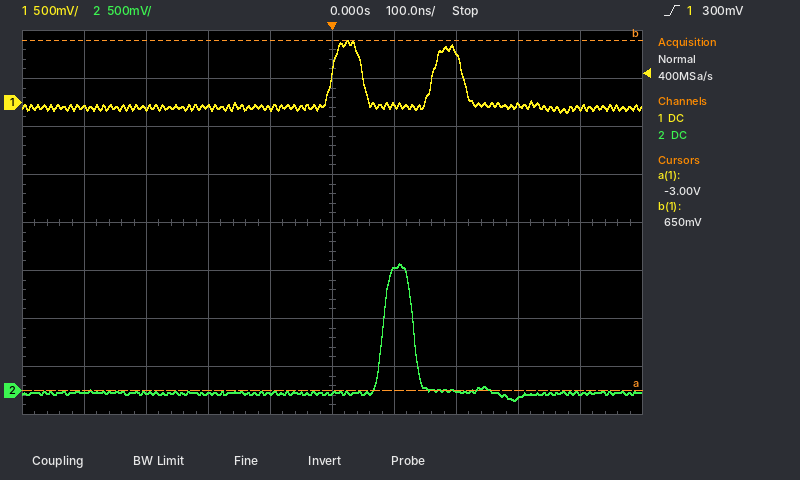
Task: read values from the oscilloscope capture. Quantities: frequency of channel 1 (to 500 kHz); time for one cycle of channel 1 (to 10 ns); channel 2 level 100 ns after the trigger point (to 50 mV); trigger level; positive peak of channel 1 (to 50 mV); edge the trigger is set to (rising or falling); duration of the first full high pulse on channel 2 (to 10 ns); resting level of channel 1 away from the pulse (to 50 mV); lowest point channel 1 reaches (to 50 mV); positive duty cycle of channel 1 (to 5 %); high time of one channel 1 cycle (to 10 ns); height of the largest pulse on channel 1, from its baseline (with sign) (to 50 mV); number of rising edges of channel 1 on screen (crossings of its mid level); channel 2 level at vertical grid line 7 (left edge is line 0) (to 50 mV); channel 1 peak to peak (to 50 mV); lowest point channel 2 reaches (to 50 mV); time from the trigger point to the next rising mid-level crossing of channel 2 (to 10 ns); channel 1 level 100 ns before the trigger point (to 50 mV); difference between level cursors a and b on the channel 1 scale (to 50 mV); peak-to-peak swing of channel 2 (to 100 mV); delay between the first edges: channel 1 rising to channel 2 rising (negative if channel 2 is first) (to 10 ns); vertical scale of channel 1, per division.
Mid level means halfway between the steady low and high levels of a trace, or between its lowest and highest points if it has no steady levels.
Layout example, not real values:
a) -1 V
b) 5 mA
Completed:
a) 6.0 MHz
b) 160 ns
c) 1.25 V
d) 300 mV
e) 650 mV
f) rising
g) 50 ns
h) -50 mV
i) -100 mV
j) 30 %
k) 50 ns
l) +700 mV
m) 2
n) 0 mV
o) 750 mV
p) -100 mV
q) 80 ns
r) -50 mV
s) 3.65 V
t) 1.40 V
u) +80 ns
v) 500 mV
